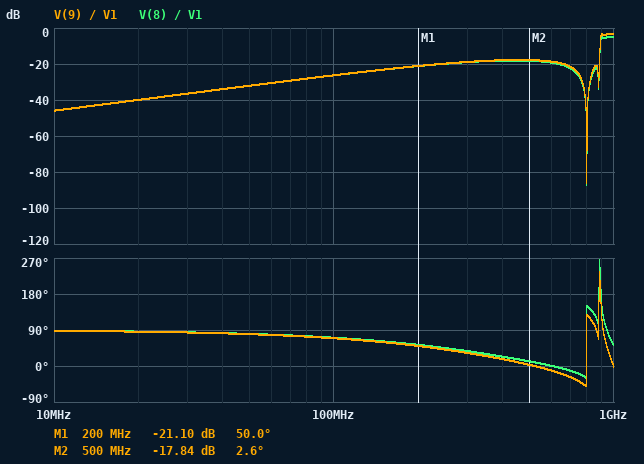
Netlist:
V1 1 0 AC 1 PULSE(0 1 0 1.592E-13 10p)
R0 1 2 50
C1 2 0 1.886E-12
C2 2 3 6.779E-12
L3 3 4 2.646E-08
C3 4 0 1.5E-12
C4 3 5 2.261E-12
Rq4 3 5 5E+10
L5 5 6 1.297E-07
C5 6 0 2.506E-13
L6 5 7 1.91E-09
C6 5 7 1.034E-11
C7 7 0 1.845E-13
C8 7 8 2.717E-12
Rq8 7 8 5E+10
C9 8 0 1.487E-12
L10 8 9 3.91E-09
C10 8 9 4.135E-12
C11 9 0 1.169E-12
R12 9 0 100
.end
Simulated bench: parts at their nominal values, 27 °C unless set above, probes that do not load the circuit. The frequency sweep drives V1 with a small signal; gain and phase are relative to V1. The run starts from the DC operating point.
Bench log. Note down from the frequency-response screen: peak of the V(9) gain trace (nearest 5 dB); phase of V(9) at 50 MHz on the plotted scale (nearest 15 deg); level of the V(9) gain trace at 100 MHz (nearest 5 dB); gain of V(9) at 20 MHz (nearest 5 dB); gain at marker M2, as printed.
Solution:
-5 dB
75 deg
-25 dB
-40 dB
-17.84 dB
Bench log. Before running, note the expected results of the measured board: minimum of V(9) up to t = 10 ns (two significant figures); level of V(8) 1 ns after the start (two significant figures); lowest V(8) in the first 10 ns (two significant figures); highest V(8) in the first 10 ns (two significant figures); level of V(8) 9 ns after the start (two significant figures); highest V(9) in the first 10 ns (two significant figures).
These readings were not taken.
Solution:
-50 mV
85 mV
-44 mV
140 mV
-18 mV
100 mV
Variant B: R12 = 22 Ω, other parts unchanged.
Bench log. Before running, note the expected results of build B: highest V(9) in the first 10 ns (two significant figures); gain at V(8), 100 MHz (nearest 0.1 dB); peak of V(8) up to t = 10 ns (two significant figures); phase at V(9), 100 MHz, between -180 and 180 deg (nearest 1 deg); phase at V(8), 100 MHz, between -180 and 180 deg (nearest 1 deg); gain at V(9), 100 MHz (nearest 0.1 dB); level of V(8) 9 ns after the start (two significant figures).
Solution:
48 mV
-39.1 dB
100 mV
80 deg
86 deg
-39.2 dB
-28 mV
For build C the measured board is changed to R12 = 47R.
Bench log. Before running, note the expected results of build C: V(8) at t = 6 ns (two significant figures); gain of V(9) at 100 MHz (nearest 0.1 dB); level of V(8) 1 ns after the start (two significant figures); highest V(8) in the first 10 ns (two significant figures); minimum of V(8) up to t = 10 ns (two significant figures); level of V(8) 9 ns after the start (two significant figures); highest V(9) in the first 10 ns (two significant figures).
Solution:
14 mV
-32.6 dB
65 mV
120 mV
-63 mV
-23 mV
74 mV
